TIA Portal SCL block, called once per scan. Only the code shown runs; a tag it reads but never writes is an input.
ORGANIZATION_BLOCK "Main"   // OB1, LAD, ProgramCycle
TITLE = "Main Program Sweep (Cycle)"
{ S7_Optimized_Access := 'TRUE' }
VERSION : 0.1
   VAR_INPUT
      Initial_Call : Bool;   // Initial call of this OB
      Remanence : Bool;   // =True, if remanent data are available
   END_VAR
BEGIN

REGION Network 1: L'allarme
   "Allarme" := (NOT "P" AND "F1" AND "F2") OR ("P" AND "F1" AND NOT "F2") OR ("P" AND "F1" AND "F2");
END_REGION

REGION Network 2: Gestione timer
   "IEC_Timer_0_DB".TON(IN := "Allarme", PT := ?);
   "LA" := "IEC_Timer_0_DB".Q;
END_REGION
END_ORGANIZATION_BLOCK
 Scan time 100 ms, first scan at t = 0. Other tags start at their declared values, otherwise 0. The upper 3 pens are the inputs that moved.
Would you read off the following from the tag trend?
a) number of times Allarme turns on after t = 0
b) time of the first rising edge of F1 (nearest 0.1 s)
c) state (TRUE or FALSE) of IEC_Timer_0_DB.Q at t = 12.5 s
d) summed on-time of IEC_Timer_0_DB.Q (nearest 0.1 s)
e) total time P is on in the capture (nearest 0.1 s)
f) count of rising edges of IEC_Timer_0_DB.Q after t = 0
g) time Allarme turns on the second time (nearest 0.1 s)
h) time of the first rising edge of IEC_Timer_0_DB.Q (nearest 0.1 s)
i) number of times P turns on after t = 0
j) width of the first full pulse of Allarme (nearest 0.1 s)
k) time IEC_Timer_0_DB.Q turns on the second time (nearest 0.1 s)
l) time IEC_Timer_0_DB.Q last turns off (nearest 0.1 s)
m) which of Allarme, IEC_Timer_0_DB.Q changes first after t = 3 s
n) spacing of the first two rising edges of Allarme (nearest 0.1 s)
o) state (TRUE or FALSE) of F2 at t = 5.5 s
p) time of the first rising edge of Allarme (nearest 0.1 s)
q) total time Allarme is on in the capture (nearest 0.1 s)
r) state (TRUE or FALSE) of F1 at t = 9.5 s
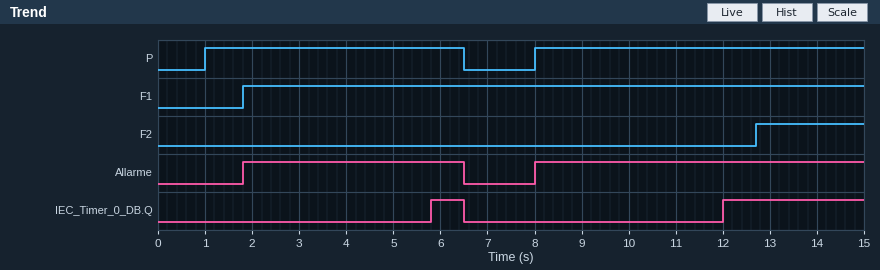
2
1.8 s
TRUE
3.7 s
12.5 s
2
8.0 s
5.8 s
2
4.7 s
12.0 s
6.5 s
IEC_Timer_0_DB.Q
6.2 s
FALSE
1.8 s
11.7 s
TRUE
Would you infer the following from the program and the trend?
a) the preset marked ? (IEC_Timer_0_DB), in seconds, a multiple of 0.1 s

4.0 s
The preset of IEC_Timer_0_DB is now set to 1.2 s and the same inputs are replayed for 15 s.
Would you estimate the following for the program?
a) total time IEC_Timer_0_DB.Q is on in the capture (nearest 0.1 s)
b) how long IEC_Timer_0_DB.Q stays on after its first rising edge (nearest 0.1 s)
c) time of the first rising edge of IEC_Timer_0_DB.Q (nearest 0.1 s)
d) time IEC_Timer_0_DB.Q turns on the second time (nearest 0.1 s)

9.3 s
3.5 s
3.0 s
9.2 s
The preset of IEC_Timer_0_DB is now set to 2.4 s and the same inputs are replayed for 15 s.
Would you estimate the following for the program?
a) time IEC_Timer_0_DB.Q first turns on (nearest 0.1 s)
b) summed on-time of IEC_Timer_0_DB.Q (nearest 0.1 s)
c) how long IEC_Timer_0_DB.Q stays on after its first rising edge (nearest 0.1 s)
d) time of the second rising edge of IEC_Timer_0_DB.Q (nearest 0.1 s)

4.2 s
6.9 s
2.3 s
10.4 s
